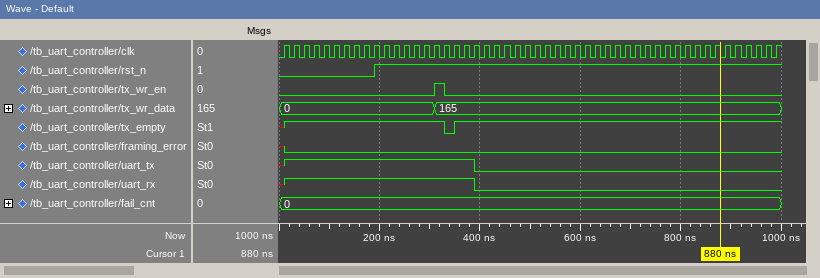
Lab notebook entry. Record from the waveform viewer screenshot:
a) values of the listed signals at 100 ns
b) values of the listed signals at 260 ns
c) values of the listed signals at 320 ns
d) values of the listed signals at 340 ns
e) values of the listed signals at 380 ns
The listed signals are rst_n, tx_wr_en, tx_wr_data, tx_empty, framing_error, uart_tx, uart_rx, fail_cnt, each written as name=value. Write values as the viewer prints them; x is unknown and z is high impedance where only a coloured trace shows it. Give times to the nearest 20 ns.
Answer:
rst_n=0, tx_wr_en=0, tx_wr_data=0, tx_empty=1, framing_error=0, uart_tx=1, uart_rx=1, fail_cnt=0
rst_n=1, tx_wr_en=0, tx_wr_data=0, tx_empty=1, framing_error=0, uart_tx=1, uart_rx=1, fail_cnt=0
rst_n=1, tx_wr_en=1, tx_wr_data=165, tx_empty=1, framing_error=0, uart_tx=1, uart_rx=1, fail_cnt=0
rst_n=1, tx_wr_en=0, tx_wr_data=165, tx_empty=0, framing_error=0, uart_tx=1, uart_rx=1, fail_cnt=0
rst_n=1, tx_wr_en=0, tx_wr_data=165, tx_empty=1, framing_error=0, uart_tx=1, uart_rx=1, fail_cnt=0
